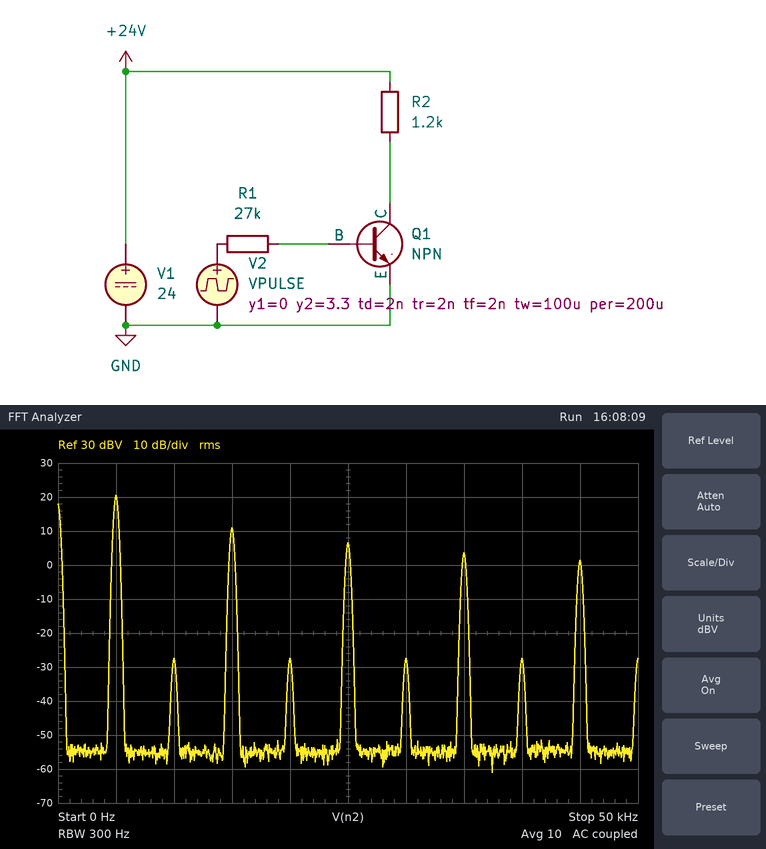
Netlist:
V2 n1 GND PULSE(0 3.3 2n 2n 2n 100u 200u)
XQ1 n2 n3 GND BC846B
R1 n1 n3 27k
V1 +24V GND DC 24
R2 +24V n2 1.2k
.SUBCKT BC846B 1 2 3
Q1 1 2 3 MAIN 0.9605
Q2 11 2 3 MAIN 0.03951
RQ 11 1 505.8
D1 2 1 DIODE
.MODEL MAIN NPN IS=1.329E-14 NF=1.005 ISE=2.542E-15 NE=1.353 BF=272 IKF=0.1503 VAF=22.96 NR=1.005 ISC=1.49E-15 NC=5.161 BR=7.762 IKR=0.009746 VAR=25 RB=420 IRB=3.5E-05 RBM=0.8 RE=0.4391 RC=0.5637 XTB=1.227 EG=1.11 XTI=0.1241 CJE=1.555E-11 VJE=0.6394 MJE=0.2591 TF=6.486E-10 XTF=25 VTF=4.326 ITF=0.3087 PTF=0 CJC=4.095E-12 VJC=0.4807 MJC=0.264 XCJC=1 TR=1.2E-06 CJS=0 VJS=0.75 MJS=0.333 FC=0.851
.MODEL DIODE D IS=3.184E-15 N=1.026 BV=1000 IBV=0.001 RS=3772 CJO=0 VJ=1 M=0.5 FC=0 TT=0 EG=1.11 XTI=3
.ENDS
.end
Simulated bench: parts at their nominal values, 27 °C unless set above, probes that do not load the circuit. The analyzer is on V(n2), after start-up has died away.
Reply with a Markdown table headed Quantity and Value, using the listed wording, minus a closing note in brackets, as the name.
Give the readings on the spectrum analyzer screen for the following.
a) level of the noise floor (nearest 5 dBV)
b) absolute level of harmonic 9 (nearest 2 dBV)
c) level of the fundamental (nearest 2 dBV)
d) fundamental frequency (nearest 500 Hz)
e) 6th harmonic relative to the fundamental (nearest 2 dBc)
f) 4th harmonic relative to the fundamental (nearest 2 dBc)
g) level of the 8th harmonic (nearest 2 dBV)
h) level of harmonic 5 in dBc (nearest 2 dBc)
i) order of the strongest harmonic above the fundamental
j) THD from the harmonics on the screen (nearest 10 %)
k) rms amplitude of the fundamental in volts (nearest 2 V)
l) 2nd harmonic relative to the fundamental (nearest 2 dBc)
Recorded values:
| Quantity | Value |
|---|---|
| level of the noise floor | -55 dBV |
| absolute level of harmonic 9 | 2 dBV |
| level of the fundamental | 20 dBV |
| fundamental frequency | 5.0 kHz |
| 6th harmonic relative to the fundamental | -48 dBc |
| 4th harmonic relative to the fundamental | -48 dBc |
| level of the 8th harmonic | -28 dBV |
| level of harmonic 5 in dBc | -14 dBc |
| order of the strongest harmonic above the fundamental | 3 |
| THD from the harmonics on the screen | 40 % |
| rms amplitude of the fundamental in volts | 10 V |
| 2nd harmonic relative to the fundamental | -48 dBc |
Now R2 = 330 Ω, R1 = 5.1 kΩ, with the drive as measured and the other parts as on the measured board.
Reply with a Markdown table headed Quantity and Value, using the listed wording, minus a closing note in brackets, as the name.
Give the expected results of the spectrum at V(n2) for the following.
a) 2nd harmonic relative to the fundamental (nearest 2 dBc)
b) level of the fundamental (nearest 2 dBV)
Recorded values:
| Quantity | Value |
|---|---|
| 2nd harmonic relative to the fundamental | -36 dBc |
| level of the fundamental | 20 dBV |
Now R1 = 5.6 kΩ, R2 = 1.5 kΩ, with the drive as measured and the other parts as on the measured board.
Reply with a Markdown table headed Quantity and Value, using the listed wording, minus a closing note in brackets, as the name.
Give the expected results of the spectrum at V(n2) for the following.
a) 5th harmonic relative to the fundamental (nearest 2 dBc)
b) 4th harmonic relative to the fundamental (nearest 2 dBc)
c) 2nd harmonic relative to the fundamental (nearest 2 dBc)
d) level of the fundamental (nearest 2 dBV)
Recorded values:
| Quantity | Value |
|---|---|
| 5th harmonic relative to the fundamental | -16 dBc |
| 4th harmonic relative to the fundamental | -18 dBc |
| 2nd harmonic relative to the fundamental | -18 dBc |
| level of the fundamental | 20 dBV |
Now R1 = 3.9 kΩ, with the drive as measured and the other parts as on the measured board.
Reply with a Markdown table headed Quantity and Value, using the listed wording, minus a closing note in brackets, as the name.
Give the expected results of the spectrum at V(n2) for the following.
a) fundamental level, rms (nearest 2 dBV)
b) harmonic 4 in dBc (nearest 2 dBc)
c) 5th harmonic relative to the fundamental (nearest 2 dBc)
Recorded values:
| Quantity | Value |
|---|---|
| fundamental level, rms | 20 dBV |
| harmonic 4 in dBc | -18 dBc |
| 5th harmonic relative to the fundamental | -16 dBc |
